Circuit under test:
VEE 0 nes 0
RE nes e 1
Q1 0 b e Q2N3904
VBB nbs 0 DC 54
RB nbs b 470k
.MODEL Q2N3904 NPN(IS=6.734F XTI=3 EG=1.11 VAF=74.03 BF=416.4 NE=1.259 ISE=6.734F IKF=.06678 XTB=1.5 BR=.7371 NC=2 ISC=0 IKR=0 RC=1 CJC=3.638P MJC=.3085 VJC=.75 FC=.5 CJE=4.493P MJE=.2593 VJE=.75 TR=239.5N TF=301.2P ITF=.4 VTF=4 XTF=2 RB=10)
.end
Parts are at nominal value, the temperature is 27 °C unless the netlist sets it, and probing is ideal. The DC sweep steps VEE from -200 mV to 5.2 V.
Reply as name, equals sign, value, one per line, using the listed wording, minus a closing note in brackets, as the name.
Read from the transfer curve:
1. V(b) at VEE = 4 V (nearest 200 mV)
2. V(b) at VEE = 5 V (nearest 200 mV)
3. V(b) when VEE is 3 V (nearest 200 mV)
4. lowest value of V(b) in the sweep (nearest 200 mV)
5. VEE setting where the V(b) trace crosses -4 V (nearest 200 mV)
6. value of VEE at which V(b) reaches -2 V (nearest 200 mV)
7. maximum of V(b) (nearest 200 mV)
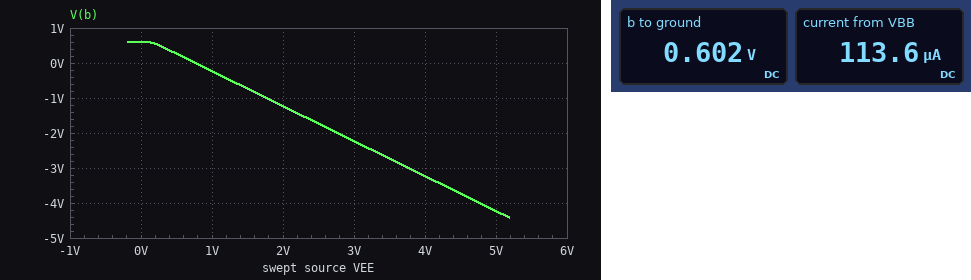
V(b) at VEE = 4 V = -3.2 V
V(b) at VEE = 5 V = -4.2 V
V(b) when VEE is 3 V = -2.2 V
lowest value of V(b) in the sweep = -4.4 V
VEE setting where the V(b) trace crosses -4 V = 4.8 V
value of VEE at which V(b) reaches -2 V = 2.8 V
maximum of V(b) = 600 mV
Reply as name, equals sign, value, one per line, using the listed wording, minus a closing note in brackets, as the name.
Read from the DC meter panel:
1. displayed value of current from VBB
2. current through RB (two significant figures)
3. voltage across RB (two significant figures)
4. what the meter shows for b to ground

displayed value of current from VBB = 113.6 µA
current through RB = 110 µA
voltage across RB = 53 V
what the meter shows for b to ground = 0.602 V
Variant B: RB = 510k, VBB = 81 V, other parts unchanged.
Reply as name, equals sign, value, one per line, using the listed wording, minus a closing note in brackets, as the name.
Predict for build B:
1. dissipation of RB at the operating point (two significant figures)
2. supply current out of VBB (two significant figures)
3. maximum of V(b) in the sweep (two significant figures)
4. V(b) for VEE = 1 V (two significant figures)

dissipation of RB at the operating point = 13 mW
supply current out of VBB = 160 µA
maximum of V(b) in the sweep = 610 mV
V(b) for VEE = 1 V = -220 mV
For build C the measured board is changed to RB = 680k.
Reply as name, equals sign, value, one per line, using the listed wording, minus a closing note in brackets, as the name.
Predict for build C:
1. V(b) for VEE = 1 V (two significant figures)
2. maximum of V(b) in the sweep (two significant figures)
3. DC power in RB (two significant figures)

V(b) for VEE = 1 V = -250 mV
maximum of V(b) in the sweep = 590 mV
DC power in RB = 4.2 mW
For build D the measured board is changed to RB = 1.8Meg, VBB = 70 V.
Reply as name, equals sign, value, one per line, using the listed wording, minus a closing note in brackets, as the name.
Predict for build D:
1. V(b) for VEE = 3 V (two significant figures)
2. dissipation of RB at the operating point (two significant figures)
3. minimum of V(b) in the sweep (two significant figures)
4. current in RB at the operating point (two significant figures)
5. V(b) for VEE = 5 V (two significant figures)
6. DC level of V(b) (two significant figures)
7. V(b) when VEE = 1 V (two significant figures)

V(b) for VEE = 3 V = -2.3 V
dissipation of RB at the operating point = 2.7 mW
minimum of V(b) in the sweep = -4.5 V
current in RB at the operating point = 39 µA
V(b) for VEE = 5 V = -4.3 V
DC level of V(b) = 570 mV
V(b) when VEE = 1 V = -280 mV
